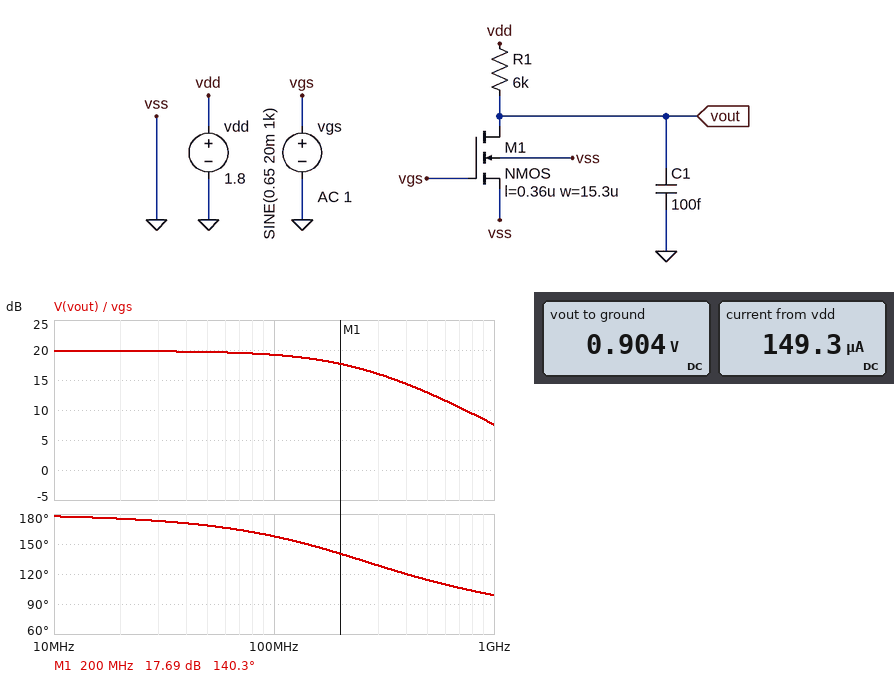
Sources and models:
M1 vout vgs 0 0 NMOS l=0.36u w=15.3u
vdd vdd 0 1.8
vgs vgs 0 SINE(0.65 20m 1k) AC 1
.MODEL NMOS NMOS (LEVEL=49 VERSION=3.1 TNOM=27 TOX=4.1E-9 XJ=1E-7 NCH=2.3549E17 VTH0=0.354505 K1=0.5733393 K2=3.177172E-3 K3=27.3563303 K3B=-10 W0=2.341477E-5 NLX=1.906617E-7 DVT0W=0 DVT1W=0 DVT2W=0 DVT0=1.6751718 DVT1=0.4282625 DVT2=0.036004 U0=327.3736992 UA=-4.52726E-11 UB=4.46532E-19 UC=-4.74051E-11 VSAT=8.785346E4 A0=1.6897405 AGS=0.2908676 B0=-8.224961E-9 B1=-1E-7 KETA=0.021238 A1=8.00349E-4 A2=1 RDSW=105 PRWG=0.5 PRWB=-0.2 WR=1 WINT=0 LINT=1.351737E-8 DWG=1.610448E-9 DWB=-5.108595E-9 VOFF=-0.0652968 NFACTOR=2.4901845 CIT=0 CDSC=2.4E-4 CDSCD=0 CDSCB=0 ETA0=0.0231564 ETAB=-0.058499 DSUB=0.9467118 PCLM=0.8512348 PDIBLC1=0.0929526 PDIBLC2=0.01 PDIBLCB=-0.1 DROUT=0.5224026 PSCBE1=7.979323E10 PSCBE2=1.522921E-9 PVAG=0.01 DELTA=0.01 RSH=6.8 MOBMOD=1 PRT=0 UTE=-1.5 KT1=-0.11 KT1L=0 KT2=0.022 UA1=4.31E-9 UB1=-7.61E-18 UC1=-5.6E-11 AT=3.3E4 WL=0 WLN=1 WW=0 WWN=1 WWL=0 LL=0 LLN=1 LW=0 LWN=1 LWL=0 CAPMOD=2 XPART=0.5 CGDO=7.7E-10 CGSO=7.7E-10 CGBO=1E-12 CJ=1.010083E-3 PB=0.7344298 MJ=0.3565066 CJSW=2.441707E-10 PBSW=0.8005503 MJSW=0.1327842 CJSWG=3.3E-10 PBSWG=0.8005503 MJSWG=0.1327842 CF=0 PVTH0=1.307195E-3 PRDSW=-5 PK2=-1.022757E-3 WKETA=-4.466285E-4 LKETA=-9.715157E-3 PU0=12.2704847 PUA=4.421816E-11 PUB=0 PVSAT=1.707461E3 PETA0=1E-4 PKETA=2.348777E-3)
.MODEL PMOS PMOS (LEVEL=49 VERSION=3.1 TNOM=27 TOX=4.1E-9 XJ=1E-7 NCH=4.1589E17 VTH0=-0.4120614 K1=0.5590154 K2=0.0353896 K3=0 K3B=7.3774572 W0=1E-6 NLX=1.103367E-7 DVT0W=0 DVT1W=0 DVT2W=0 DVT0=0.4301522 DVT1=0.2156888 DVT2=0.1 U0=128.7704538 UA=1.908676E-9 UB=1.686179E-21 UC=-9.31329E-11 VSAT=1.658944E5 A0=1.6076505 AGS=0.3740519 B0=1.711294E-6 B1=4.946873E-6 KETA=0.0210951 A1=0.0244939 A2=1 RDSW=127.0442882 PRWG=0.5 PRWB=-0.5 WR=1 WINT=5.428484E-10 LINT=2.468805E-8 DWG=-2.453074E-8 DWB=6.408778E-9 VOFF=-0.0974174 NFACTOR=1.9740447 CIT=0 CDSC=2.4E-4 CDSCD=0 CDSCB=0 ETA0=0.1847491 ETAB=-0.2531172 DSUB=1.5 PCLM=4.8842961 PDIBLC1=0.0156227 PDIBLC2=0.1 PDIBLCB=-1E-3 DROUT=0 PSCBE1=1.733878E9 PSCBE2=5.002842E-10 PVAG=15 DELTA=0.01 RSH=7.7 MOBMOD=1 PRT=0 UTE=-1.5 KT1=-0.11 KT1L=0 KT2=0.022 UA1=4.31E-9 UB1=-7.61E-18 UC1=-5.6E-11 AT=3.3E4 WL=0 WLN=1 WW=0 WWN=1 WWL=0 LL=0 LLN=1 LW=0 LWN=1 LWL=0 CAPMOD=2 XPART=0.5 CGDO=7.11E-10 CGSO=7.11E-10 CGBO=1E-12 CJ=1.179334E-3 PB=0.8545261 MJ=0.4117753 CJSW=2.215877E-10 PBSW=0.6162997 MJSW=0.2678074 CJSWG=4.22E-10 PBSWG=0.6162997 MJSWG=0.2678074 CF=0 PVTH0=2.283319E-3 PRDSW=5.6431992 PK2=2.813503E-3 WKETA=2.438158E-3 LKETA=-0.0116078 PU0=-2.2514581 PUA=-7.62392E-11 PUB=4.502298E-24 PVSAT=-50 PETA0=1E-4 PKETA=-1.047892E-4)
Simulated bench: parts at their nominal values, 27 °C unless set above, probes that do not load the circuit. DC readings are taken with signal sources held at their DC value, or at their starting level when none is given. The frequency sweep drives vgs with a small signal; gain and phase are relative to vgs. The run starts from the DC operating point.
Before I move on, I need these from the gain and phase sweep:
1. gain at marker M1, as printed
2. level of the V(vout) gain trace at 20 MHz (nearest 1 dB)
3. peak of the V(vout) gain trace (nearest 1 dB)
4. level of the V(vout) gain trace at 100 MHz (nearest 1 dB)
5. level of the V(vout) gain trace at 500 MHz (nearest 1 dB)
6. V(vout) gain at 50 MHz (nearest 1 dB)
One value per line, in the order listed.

17.69 dB
20 dB
20 dB
19 dB
13 dB
20 dB
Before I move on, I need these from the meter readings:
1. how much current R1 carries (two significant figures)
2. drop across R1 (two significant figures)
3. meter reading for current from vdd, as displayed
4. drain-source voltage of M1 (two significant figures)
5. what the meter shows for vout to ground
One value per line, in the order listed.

150 µA
900 mV
149.3 µA
900 mV
0.904 V
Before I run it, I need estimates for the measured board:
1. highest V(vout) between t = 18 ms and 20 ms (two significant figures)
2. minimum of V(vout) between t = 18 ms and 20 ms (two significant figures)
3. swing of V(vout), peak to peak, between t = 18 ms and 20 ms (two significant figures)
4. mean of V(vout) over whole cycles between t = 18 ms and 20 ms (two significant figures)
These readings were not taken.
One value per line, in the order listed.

1.1 V
700 mV
390 mV
900 mV
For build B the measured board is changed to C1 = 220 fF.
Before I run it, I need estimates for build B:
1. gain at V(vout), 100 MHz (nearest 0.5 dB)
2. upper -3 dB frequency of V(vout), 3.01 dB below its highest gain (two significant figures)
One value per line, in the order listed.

17.5 dB
120 MHz
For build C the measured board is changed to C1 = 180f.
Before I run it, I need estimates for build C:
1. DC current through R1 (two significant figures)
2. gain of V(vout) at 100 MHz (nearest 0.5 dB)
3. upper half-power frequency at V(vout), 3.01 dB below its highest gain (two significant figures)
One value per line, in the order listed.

150 µA
18.0 dB
150 MHz
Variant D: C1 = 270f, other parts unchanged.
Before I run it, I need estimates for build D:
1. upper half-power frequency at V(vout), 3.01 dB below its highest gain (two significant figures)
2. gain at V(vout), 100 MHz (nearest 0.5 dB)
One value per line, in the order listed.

100 MHz
17.0 dB
